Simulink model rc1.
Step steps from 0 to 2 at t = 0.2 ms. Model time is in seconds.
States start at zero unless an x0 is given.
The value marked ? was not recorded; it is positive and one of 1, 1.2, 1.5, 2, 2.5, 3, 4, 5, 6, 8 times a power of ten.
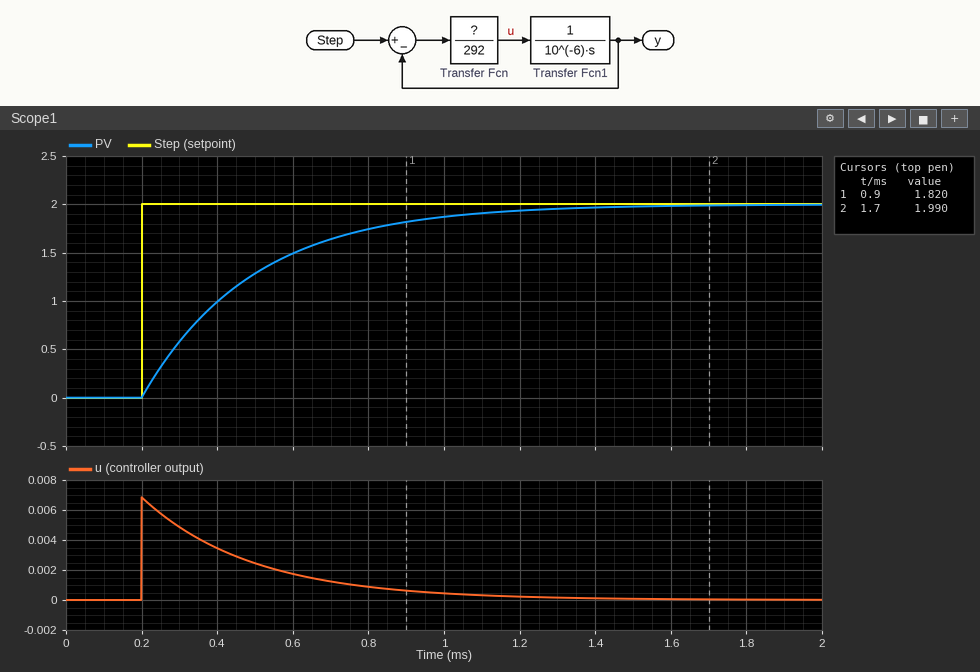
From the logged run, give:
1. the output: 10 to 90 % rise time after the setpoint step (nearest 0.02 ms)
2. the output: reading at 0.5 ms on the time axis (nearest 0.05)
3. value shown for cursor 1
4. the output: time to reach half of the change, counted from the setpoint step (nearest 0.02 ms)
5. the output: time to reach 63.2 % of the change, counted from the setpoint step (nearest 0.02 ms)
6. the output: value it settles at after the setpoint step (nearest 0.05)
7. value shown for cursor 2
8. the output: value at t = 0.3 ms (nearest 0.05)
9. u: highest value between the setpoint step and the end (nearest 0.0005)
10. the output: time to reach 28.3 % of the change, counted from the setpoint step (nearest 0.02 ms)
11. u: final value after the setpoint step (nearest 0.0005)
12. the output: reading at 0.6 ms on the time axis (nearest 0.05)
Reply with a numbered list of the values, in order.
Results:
1. 0.64 ms
2. 1.30
3. 1.820
4. 0.20 ms
5. 0.30 ms
6. 2.00
7. 1.990
8. 0.60
9. 0.0070
10. 0.10 ms
11. 0.0000
12. 1.50
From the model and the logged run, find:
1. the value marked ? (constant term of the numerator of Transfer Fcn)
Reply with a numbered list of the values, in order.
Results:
1. 1
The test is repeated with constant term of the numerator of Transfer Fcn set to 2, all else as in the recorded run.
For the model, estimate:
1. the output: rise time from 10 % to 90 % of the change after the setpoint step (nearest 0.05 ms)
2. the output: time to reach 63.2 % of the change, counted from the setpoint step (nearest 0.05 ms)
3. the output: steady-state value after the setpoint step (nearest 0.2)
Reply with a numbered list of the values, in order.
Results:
1. 0.30 ms
2. 0.15 ms
3. 2.0
